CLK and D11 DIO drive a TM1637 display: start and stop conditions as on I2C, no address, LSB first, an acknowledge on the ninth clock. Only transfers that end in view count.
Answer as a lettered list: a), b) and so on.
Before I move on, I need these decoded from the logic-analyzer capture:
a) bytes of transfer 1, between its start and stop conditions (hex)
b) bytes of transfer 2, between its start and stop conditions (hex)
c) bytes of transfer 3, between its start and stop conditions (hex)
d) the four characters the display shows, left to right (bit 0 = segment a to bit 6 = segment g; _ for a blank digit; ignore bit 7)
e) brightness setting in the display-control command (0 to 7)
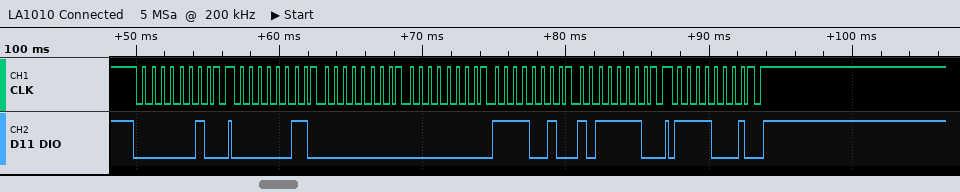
a) 40
b) C0 00 00 4F 7D
c) 8F
d) __36
e) 7
